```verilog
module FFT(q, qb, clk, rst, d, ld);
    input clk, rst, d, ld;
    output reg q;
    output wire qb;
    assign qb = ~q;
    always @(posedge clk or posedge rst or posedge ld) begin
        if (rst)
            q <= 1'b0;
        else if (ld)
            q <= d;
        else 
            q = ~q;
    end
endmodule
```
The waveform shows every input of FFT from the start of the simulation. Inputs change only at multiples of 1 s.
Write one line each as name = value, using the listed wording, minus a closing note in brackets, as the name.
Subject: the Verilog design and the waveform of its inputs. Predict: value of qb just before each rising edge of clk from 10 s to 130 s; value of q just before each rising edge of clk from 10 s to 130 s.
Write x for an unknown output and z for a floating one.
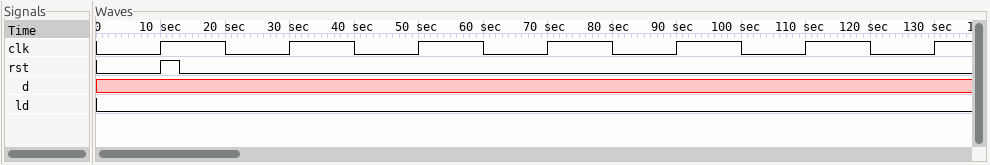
value of qb just before each rising edge of clk from 10 s to 130 s = x 1 0 1 0 1 0
value of q just before each rising edge of clk from 10 s to 130 s = x 0 1 0 1 0 1
